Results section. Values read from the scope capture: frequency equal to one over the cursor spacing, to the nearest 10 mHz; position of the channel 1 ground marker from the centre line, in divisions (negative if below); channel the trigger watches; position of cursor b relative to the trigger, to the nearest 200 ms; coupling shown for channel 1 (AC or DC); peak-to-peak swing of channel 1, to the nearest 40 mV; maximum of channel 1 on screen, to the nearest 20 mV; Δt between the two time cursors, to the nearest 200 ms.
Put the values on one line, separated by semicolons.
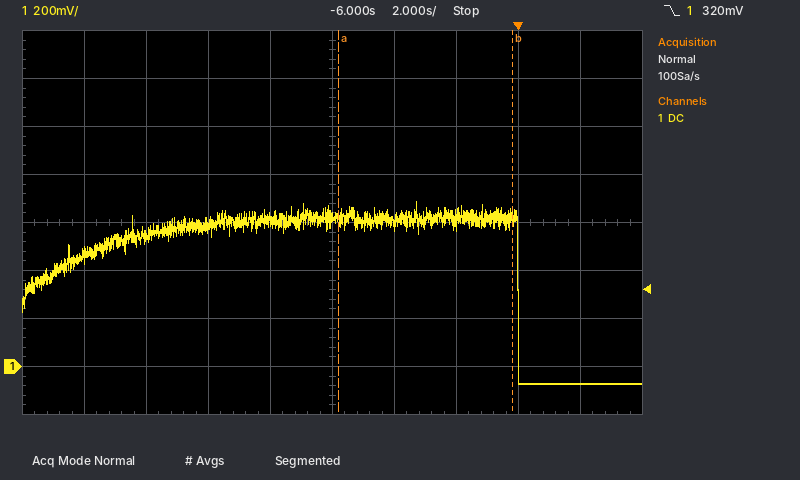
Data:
180 mHz; -3.0 div; channel 1; -200 ms; DC; 760 mV; 680 mV; 5.6 s
